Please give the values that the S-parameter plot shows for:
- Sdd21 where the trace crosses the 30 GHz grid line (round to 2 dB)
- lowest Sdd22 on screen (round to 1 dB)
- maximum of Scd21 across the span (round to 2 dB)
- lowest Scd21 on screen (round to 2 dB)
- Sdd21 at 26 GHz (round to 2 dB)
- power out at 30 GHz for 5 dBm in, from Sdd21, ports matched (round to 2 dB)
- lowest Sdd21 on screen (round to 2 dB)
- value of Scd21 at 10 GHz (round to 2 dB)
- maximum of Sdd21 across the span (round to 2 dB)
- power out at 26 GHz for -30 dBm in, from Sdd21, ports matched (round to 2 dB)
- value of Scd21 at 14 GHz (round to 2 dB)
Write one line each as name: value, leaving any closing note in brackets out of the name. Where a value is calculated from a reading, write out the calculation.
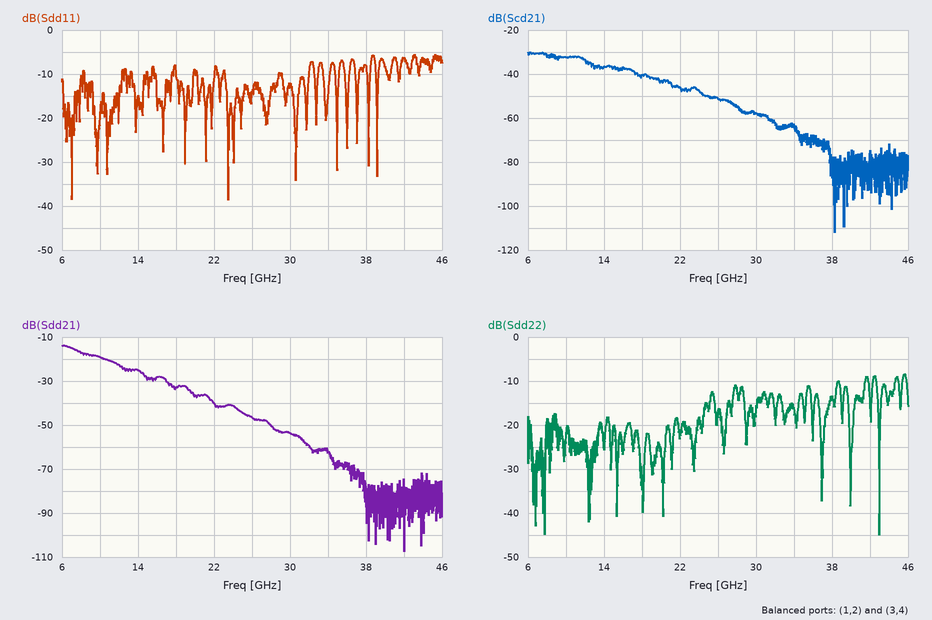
Sdd21 where the trace crosses the 30 GHz grid line: -54 dB
lowest Sdd22 on screen: -45 dB
maximum of Scd21 across the span: -30 dB
lowest Scd21 on screen: -112 dB
Sdd21 at 26 GHz: -46 dB
power out at 30 GHz for 5 dBm in, from Sdd21, ports matched: 5 dBm + (-54 dB) = -48 dBm
lowest Sdd21 on screen: -108 dB
value of Scd21 at 10 GHz: -32 dB
maximum of Sdd21 across the span: -14 dB
power out at 26 GHz for -30 dBm in, from Sdd21, ports matched: -30 dBm + (-46 dB) = -76 dBm
value of Scd21 at 14 GHz: -36 dB
